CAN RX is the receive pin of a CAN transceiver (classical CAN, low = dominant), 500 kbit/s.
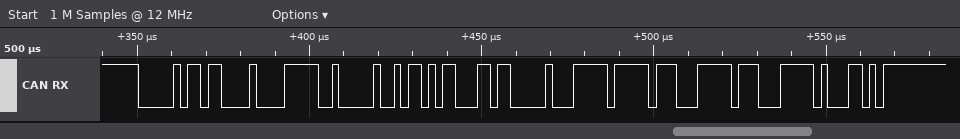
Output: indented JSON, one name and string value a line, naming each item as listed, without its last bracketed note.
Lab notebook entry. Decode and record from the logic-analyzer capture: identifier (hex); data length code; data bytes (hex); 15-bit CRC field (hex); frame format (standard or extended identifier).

{
  "identifier": "0x036",
  "data length code": "8",
  "data bytes": "7D 01 6B 1B 00 FF F8 FF",
  "15-bit CRC field": "0x0FC6",
  "frame format": "standard"
}
